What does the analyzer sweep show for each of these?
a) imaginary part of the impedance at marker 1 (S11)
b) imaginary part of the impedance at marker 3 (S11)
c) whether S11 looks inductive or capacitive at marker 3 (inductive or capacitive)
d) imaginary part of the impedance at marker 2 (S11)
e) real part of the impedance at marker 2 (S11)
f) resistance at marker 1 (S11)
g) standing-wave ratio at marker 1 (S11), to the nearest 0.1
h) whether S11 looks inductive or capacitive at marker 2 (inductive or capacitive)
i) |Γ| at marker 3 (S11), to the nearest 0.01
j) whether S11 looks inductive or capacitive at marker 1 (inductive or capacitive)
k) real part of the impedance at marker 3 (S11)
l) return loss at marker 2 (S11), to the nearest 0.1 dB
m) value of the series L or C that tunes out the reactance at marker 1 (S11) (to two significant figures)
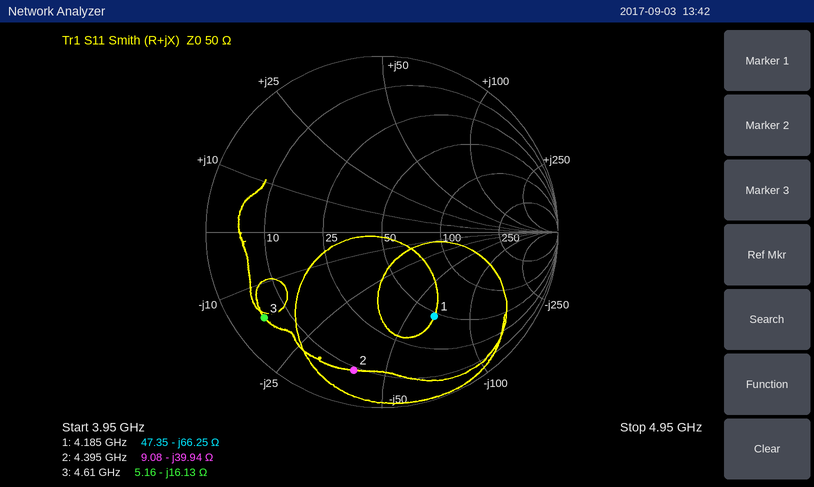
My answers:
-66.25 Ω
-16.13 Ω
capacitive
-39.94 Ω
9.08 Ω
47.35 Ω
3.6
capacitive
0.83
capacitive
5.16 Ω
1.9 dB
2.5 nH
